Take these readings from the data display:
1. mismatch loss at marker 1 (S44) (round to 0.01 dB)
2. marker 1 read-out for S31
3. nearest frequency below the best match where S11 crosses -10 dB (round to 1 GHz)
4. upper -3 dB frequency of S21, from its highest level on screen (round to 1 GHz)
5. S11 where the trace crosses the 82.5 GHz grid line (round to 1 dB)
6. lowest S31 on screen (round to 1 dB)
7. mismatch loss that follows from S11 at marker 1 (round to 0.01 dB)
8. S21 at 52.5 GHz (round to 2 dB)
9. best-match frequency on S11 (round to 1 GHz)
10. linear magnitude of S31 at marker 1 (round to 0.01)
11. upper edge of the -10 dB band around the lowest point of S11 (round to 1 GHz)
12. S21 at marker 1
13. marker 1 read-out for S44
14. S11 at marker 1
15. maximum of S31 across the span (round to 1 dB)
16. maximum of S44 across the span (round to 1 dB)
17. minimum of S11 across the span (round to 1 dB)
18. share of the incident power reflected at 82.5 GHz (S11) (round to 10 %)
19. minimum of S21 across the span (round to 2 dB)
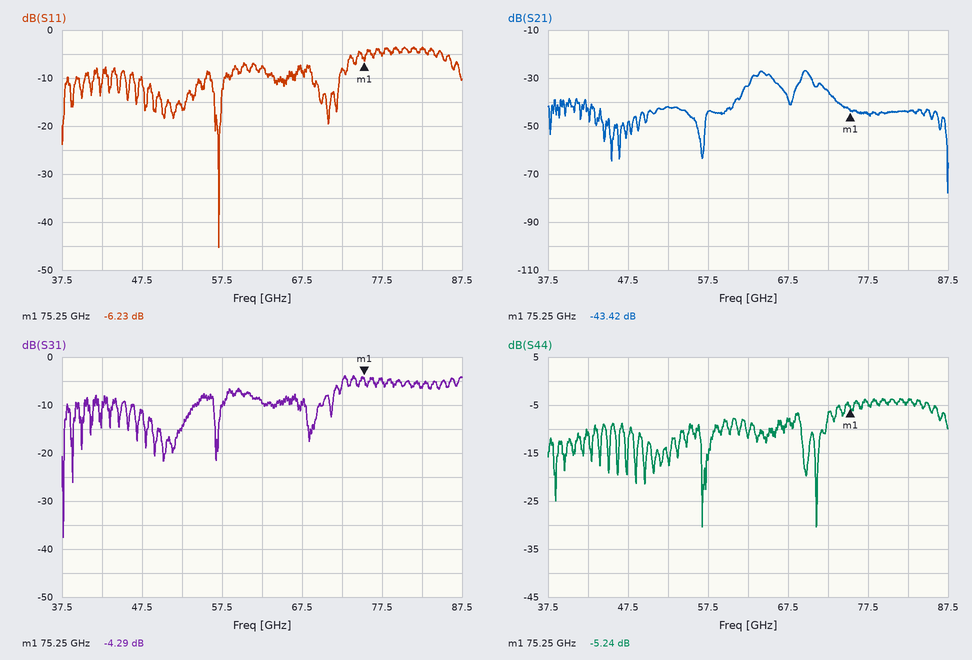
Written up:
1.54 dB
-4.29 dB
56 GHz
70 GHz
-4 dB
-38 dB
1.18 dB
-42 dB
57 GHz
0.61
58 GHz
-43.42 dB
-5.24 dB
-6.23 dB
-4 dB
-4 dB
-45 dB
40 %
-78 dB
